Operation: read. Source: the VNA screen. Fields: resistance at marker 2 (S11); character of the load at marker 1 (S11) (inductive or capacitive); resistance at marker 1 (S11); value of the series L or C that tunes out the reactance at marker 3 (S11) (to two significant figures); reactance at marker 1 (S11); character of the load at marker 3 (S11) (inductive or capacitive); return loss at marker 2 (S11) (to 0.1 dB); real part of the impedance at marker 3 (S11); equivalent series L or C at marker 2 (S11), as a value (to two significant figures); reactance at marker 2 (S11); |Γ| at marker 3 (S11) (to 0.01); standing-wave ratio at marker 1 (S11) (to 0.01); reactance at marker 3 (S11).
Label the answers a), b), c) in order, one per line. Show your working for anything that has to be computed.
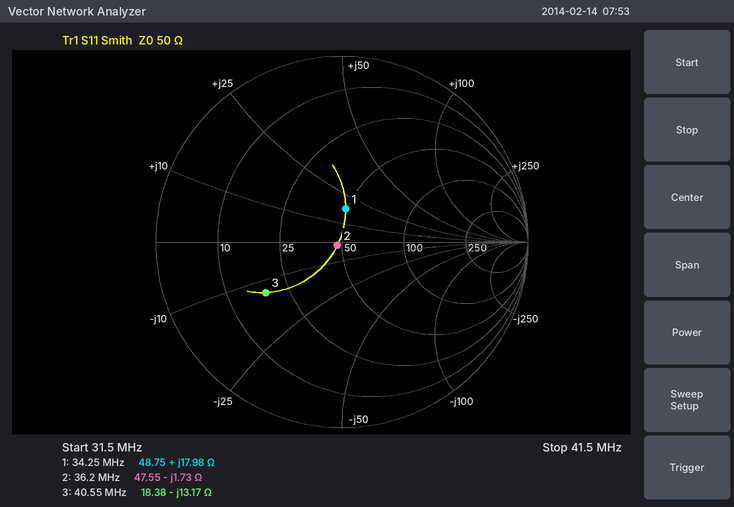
a) 47.55 Ω
b) inductive
c) 48.75 Ω
d) L = 13.17 Ω/(2π × 40.55 MHz) ≈ 52 nH
e) +17.98 Ω
f) capacitive
g) 30.2 dB
h) 18.38 Ω
i) C = 1/(2π × 36.2 MHz × 1.73 Ω) ≈ 2.5 nF
j) -1.73 Ω
k) 0.49
l) 1.44
m) -13.17 Ω
